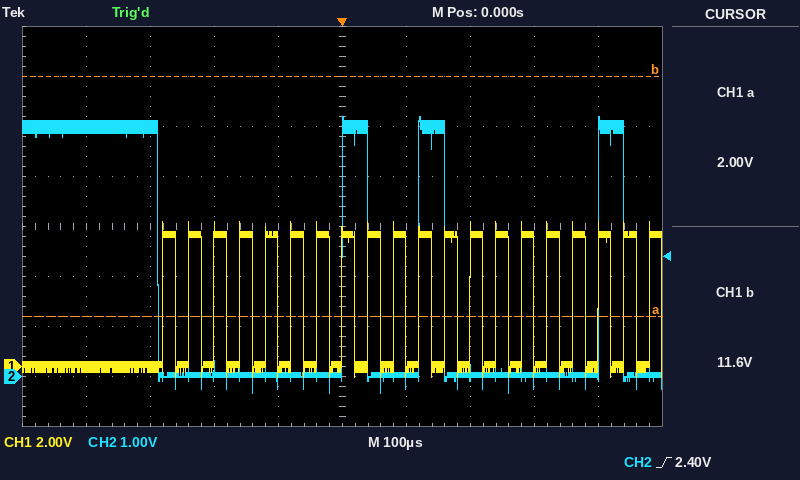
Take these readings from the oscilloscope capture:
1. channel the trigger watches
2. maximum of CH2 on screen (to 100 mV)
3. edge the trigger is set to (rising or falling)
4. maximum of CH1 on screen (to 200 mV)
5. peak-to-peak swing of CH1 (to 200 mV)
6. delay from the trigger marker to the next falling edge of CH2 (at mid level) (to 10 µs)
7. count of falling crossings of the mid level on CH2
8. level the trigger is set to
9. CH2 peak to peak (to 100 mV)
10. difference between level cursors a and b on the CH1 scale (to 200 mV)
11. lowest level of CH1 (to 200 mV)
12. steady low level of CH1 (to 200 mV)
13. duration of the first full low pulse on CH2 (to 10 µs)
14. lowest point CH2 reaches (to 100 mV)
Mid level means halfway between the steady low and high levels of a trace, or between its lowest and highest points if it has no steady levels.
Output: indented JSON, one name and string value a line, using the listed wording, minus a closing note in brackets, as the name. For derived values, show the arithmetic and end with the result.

{
  "channel the trigger watches": "CH2",
  "maximum of CH2 on screen": "5.2 V",
  "edge the trigger is set to": "rising",
  "maximum of CH1 on screen": "5.8 V",
  "peak-to-peak swing of CH1": "5.8 V − (-400 mV) = 6.2 V",
  "delay from the trigger marker to the next falling edge of CH2 (at mid level)": "40 µs",
  "count of falling crossings of the mid level on CH2": "4",
  "level the trigger is set to": "2.40 V",
  "CH2 peak to peak": "5.2 V − (-300 mV) = 5.5 V",
  "difference between level cursors a and b on the CH1 scale": "9.6 V",
  "lowest level of CH1": "-400 mV",
  "steady low level of CH1": "0.0 V",
  "duration of the first full low pulse on CH2": "290 µs",
  "lowest point CH2 reaches": "-300 mV"
}
